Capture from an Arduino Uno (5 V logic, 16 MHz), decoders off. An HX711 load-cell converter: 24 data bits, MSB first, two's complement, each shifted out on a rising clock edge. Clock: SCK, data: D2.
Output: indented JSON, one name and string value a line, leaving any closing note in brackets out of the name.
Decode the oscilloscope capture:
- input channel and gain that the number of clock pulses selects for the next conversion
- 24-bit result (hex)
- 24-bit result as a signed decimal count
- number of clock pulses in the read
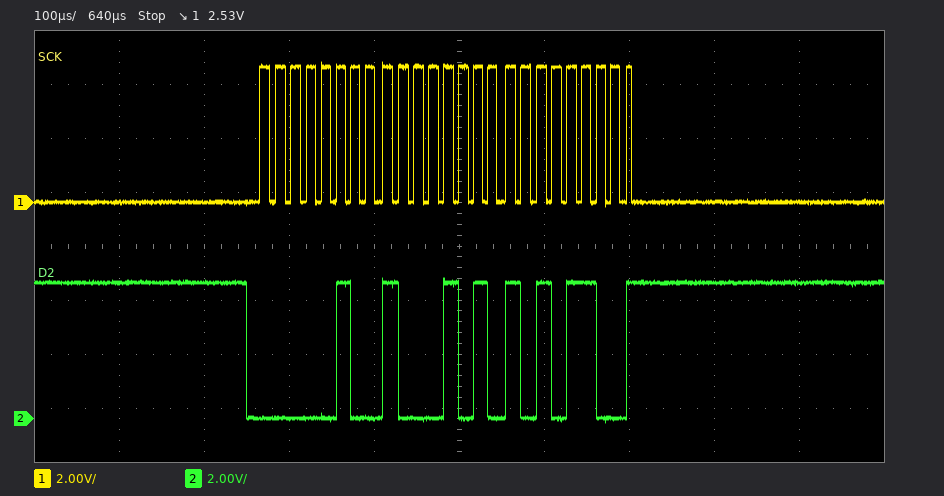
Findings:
{
  "input channel and gain that the number of clock pulses selects for the next conversion": "channel A, gain 128",
  "24-bit result": "0x048AAC",
  "24-bit result as a signed decimal count": "297644",
  "number of clock pulses in the read": "25"
}
